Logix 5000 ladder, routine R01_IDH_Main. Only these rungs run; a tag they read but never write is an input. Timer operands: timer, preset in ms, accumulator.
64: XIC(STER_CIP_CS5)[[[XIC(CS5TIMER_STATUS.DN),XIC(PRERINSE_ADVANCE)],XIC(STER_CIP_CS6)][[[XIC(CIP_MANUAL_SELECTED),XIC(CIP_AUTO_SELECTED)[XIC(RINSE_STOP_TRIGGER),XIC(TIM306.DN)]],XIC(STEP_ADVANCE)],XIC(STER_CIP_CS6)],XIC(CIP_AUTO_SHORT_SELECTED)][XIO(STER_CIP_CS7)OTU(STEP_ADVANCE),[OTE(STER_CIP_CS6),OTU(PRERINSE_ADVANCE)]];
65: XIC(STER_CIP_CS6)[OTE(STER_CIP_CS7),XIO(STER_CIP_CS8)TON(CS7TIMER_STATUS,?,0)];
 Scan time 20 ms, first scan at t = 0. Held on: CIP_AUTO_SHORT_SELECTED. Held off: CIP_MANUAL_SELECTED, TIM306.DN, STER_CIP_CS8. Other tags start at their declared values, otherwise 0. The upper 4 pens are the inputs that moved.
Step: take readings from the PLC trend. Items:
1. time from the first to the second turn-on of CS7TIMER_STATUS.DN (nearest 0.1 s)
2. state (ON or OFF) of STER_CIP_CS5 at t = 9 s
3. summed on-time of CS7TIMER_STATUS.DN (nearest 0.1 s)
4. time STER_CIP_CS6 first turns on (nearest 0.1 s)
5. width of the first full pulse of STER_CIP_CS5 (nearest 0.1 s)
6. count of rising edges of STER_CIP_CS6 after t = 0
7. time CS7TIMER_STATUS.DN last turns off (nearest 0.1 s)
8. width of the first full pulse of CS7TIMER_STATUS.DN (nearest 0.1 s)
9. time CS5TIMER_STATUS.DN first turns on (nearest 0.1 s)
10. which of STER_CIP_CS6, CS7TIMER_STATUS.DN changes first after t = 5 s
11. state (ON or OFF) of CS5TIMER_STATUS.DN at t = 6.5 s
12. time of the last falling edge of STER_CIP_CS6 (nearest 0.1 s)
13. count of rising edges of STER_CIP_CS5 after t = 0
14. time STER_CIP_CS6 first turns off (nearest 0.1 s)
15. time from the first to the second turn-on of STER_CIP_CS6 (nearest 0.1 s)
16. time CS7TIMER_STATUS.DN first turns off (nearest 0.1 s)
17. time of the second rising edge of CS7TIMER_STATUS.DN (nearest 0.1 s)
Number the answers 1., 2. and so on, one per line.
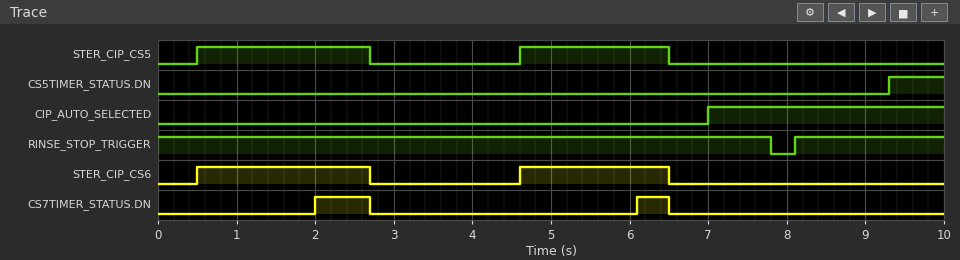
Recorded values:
1. 4.1 s
2. OFF
3. 1.1 s
4. 0.5 s
5. 2.2 s
6. 2
7. 6.5 s
8. 0.7 s
9. 9.3 s
10. CS7TIMER_STATUS.DN
11. OFF
12. 6.5 s
13. 2
14. 2.7 s
15. 4.1 s
16. 2.7 s
17. 6.1 s
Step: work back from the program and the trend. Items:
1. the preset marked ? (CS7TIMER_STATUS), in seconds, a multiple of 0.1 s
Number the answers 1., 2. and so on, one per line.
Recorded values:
1. 1.5 s
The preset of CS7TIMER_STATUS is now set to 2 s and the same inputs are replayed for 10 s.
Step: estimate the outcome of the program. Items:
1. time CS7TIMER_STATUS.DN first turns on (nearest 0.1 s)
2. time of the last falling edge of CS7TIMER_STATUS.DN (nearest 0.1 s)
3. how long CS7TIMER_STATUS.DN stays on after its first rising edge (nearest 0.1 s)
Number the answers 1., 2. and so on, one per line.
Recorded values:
1. 2.5 s
2. 2.7 s
3. 0.2 s
